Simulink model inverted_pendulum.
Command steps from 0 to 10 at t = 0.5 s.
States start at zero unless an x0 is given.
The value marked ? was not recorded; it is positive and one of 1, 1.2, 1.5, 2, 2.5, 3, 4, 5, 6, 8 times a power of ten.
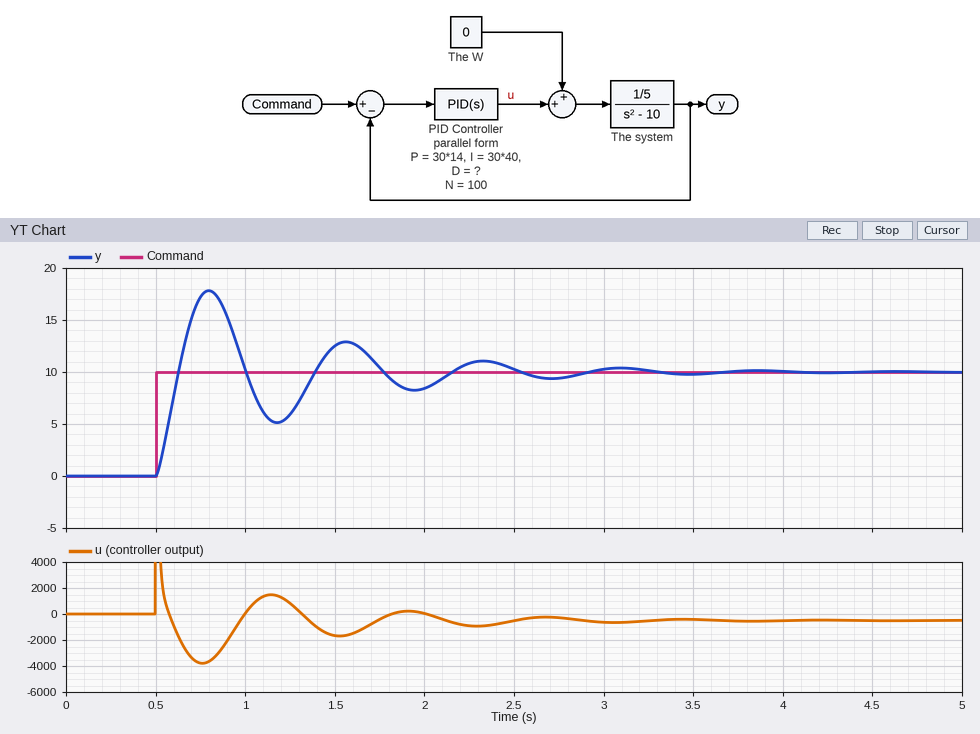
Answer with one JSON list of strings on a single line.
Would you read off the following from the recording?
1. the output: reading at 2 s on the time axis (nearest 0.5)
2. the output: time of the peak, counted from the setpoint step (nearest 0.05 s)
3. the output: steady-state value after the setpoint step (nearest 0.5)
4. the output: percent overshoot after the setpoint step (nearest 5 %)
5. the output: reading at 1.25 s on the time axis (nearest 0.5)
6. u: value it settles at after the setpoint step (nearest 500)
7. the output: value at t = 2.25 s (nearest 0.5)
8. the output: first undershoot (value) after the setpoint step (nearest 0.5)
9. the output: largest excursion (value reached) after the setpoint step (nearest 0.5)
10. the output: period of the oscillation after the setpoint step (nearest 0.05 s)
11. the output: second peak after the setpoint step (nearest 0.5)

["8.5", "0.30 s", "10.0", "80 %", "6.0", "-500", "11.0", "5.0", "18.0", "0.75 s", "13.0"]
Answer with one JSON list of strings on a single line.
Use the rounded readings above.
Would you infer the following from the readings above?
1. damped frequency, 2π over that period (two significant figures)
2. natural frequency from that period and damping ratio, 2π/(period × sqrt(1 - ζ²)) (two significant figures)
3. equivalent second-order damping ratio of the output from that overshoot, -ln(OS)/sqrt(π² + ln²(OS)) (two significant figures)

["8.4 rad/s", "8.4 rad/s", "0.071"]
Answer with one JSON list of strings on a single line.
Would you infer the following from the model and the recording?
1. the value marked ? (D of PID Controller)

["30"]
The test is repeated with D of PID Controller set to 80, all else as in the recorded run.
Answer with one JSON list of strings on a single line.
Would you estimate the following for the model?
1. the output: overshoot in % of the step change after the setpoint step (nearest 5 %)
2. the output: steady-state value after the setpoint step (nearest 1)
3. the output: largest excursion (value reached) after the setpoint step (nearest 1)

["30 %", "10", "13"]
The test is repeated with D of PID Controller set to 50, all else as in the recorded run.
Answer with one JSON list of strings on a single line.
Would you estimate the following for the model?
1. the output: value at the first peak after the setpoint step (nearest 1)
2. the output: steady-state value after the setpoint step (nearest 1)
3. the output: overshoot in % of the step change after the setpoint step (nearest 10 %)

["15", "10", "50 %"]
